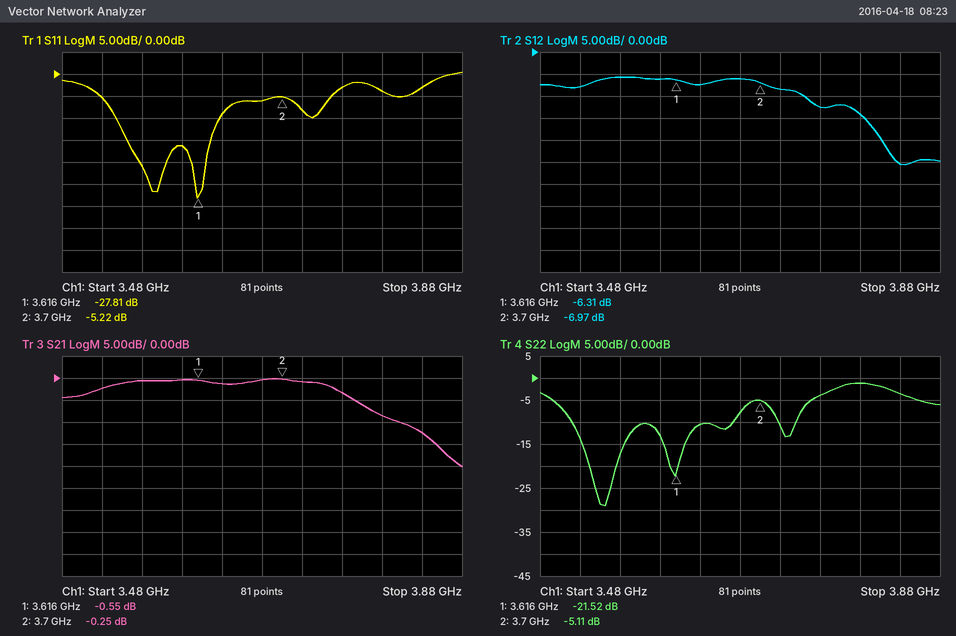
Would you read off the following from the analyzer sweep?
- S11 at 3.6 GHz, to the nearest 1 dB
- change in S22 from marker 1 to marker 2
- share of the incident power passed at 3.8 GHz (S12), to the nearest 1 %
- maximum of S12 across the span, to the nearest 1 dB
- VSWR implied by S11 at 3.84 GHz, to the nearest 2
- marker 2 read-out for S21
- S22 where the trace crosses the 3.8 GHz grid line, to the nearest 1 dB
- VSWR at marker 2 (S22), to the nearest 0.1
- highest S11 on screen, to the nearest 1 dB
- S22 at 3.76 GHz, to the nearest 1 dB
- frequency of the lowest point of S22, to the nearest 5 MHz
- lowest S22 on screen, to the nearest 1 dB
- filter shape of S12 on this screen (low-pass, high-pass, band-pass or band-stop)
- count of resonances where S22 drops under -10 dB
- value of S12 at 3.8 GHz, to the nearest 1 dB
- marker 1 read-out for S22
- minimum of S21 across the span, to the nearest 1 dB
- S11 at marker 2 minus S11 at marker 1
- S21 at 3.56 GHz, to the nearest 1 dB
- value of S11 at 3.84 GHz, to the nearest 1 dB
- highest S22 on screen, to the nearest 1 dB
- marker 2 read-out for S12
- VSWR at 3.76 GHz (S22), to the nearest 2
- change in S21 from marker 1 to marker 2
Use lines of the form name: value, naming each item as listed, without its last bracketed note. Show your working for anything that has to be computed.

S11 at 3.6 GHz, to the nearest 1 dB: -16 dB
change in S22 from marker 1 to marker 2: -5.11 − (-21.52) = 16.41 dB
share of the incident power passed at 3.8 GHz (S12), to the nearest 1 %: 10^(-14/10) ≈ 4 %
maximum of S12 across the span, to the nearest 1 dB: -6 dB
VSWR implied by S11 at 3.84 GHz, to the nearest 2: |Γ| = 10^(-3/20) = 0.7079; VSWR = (1 + 0.7079)/(1 − 0.7079) ≈ 6
marker 2 read-out for S21: -0.25 dB
S22 where the trace crosses the 3.8 GHz grid line, to the nearest 1 dB: -1 dB
VSWR at marker 2 (S22), to the nearest 0.1: (1 + 0.5553)/(1 − 0.5553) ≈ 3.5
highest S11 on screen, to the nearest 1 dB: 0 dB
S22 at 3.76 GHz, to the nearest 1 dB: -4 dB
frequency of the lowest point of S22, to the nearest 5 MHz: 3.545 GHz
lowest S22 on screen, to the nearest 1 dB: -29 dB
filter shape of S12 on this screen: low-pass
count of resonances where S22 drops under -10 dB: 3
value of S12 at 3.8 GHz, to the nearest 1 dB: -14 dB
marker 1 read-out for S22: -21.52 dB
minimum of S21 across the span, to the nearest 1 dB: -20 dB
S11 at marker 2 minus S11 at marker 1: -5.22 − (-27.81) = 22.59 dB
S21 at 3.56 GHz, to the nearest 1 dB: -1 dB
value of S11 at 3.84 GHz, to the nearest 1 dB: -3 dB
highest S22 on screen, to the nearest 1 dB: -1 dB
marker 2 read-out for S12: -6.97 dB
VSWR at 3.76 GHz (S22), to the nearest 2: |Γ| = 10^(-4/20) = 0.6310; VSWR = (1 + 0.6310)/(1 − 0.6310) ≈ 4
change in S21 from marker 1 to marker 2: -0.25 − (-0.55) = 0.30 dB
